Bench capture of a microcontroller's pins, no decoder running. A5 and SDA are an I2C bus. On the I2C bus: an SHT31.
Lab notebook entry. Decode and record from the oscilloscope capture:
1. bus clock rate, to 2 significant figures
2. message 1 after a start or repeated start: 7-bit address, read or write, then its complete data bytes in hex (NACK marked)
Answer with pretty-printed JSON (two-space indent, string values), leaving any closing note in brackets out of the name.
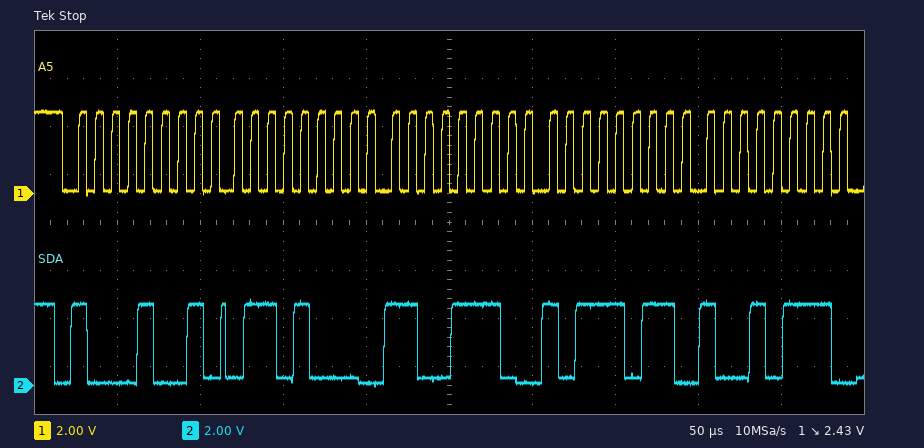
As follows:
{
  "bus clock rate, to 2 significant figures": "100 kHz",
  "message 1 after a start or repeated start: 7-bit address, read or write, then its complete data bytes in hex": "0x44 read: 68 CE BB 97"
}
